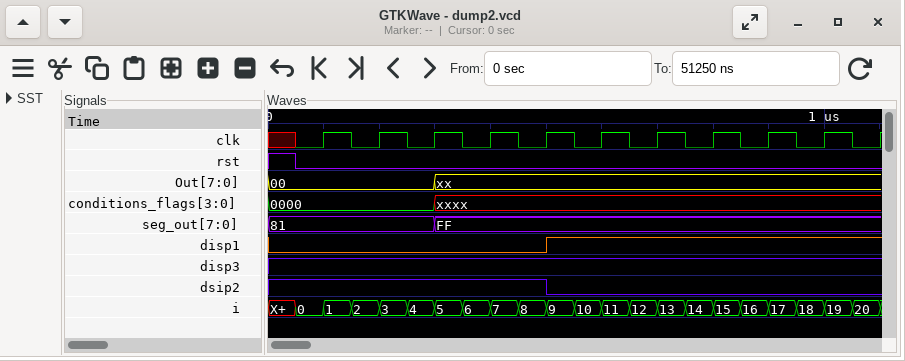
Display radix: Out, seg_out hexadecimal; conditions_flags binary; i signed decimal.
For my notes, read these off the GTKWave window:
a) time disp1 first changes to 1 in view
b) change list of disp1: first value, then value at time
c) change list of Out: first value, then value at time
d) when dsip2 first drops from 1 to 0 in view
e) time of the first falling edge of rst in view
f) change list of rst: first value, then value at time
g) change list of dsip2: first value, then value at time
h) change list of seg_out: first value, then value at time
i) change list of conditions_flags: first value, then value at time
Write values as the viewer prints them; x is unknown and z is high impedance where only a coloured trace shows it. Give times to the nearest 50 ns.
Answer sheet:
500 ns
0, 1 at 500 ns
00, xx at 300 ns
500 ns
50 ns
1, 0 at 50 ns
1, 0 at 500 ns
81, FF at 300 ns
0000, xxxx at 300 ns
